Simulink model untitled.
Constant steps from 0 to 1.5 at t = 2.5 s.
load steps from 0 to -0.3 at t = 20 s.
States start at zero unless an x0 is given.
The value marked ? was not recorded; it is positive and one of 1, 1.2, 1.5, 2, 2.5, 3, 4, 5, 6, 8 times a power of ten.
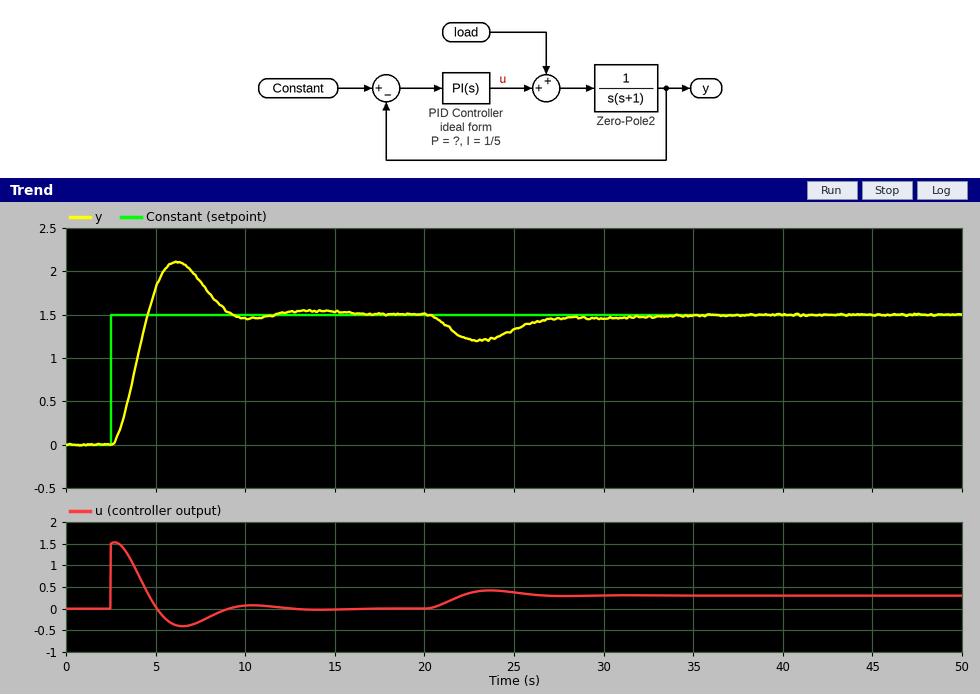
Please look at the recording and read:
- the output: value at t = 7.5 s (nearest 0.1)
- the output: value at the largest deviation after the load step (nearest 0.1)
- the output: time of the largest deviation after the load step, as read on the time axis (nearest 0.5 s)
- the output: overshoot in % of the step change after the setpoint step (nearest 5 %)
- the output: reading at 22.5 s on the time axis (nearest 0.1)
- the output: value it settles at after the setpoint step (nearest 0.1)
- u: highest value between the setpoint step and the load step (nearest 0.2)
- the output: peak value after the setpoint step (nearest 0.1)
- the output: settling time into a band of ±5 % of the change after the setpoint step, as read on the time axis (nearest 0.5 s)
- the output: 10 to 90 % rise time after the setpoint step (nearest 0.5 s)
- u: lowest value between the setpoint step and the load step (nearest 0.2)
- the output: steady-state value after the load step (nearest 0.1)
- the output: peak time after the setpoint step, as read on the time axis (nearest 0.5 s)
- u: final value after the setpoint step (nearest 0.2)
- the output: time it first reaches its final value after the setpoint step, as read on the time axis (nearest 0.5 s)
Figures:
1.9
1.2
23.0 s
40 %
1.2
1.5
1.6
2.1
9.0 s
1.5 s
-0.4
1.5
6.0 s
0.0
4.5 s
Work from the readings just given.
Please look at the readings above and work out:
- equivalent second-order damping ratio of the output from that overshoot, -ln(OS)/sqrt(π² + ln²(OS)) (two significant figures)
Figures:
0.28
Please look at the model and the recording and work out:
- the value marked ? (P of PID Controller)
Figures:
1
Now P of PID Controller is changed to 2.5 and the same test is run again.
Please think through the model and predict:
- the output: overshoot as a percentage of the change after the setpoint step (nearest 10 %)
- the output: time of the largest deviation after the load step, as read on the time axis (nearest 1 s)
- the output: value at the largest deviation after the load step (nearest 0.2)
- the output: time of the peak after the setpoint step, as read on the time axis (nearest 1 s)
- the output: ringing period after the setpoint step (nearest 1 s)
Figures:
50 %
22 s
1.4
5 s
4 s
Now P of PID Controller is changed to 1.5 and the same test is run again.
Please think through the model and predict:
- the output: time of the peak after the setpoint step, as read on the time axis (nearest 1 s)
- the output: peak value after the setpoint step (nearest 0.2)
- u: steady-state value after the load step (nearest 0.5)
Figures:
5 s
2.2
0.5
